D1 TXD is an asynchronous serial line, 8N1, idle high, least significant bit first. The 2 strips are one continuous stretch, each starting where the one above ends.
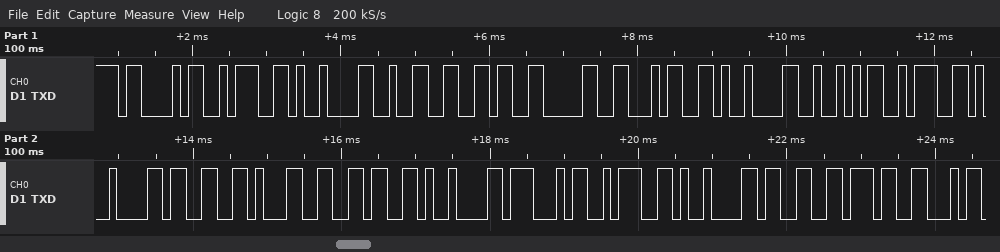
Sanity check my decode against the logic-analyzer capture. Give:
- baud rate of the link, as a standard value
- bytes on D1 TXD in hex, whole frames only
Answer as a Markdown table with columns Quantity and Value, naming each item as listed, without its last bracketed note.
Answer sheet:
| Quantity | Value |
|---|---|
| baud rate of the link, as a standard value | 9600 baud |
| bytes on D1 TXD in hex, whole frames only | 43 3A 09 32 36 30 34 09 52 3A 09 33 31 36 09 47 3A 09 33 37 |
